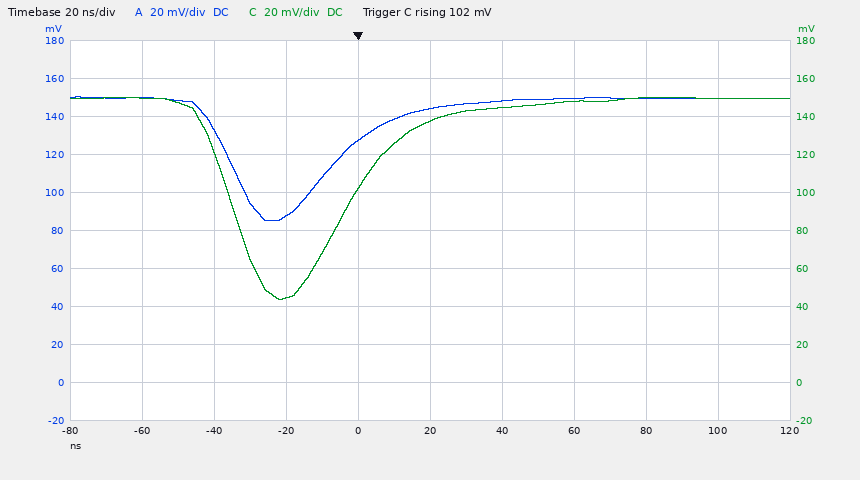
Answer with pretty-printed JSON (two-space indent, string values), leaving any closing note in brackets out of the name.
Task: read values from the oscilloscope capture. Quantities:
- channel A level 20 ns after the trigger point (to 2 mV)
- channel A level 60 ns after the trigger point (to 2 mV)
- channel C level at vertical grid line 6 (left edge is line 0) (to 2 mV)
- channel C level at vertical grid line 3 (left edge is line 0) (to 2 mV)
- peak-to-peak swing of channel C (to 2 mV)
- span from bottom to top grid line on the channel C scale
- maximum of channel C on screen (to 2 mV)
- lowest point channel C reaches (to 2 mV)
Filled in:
{
  "channel A level 20 ns after the trigger point": "144 mV",
  "channel A level 60 ns after the trigger point": "150 mV",
  "channel C level at vertical grid line 6 (left edge is line 0)": "144 mV",
  "channel C level at vertical grid line 3 (left edge is line 0)": "44 mV",
  "peak-to-peak swing of channel C": "106 mV",
  "span from bottom to top grid line on the channel C scale": "200 mV",
  "maximum of channel C on screen": "150 mV",
  "lowest point channel C reaches": "44 mV"
}
